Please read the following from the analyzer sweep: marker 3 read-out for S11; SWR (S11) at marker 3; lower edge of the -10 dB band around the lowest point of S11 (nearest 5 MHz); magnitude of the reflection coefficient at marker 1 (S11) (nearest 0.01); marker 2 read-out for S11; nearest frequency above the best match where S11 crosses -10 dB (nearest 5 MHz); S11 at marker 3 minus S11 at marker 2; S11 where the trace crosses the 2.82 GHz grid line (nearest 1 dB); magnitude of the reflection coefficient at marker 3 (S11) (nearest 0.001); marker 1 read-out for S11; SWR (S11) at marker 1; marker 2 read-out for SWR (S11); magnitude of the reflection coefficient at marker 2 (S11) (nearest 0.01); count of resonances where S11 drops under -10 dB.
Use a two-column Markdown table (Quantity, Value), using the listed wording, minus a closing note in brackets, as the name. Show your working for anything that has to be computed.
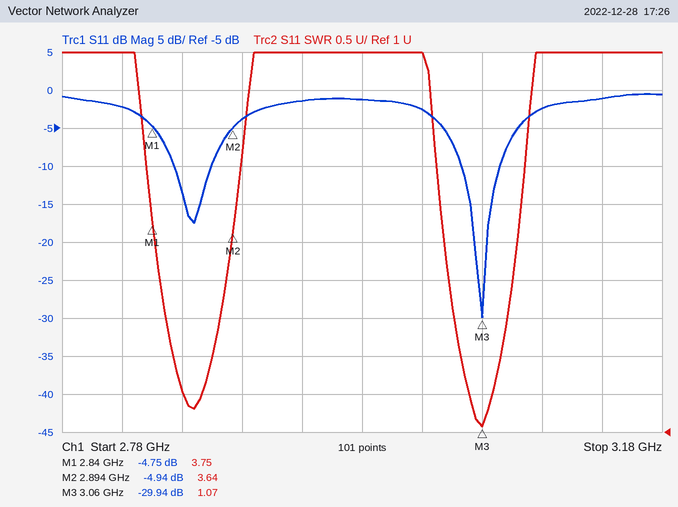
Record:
| Quantity | Value |
|---|---|
| marker 3 read-out for S11 | -29.94 dB |
| SWR (S11) at marker 3 | 1.07 |
| lower edge of the -10 dB band around the lowest point of S11 | 3.045 GHz |
| magnitude of the reflection coefficient at marker 1 (S11) | 10^(-4.75/20) ≈ 0.58 |
| marker 2 read-out for S11 | -4.94 dB |
| nearest frequency above the best match where S11 crosses -10 dB | 3.070 GHz |
| S11 at marker 3 minus S11 at marker 2 | -29.94 − (-4.94) = -25.00 dB |
| S11 where the trace crosses the 2.82 GHz grid line | -2 dB |
| magnitude of the reflection coefficient at marker 3 (S11) | 10^(-29.94/20) ≈ 0.032 |
| marker 1 read-out for S11 | -4.75 dB |
| SWR (S11) at marker 1 | 3.75 |
| marker 2 read-out for SWR | 3.64 |
| magnitude of the reflection coefficient at marker 2 (S11) | 10^(-4.94/20) ≈ 0.57 |
| count of resonances where S11 drops under -10 dB | 2 |
